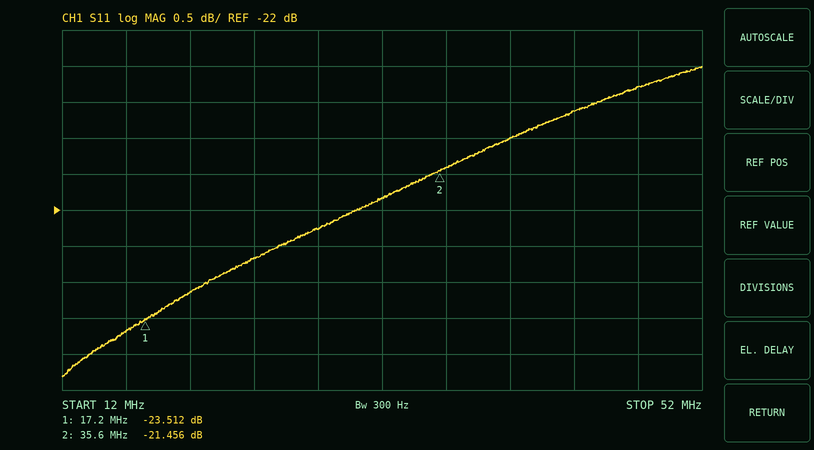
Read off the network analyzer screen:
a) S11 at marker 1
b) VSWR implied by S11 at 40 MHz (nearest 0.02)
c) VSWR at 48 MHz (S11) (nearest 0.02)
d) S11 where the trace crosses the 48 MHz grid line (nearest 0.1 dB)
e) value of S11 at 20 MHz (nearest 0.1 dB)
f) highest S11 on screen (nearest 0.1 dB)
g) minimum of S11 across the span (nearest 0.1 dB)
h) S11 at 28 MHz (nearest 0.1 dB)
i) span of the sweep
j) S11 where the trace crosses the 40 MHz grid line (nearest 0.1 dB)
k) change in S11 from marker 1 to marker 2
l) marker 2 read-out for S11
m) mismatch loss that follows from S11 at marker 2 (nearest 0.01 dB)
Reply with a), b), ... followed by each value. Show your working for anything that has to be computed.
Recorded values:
a) -23.512 dB
b) |Γ| = 10^(-21/20) = 0.0891; VSWR = (1 + 0.0891)/(1 − 0.0891) ≈ 1.20
c) |Γ| = 10^(-20.3/20) = 0.0966; VSWR = (1 + 0.0966)/(1 − 0.0966) ≈ 1.21, so 1.22 to the nearest 0.02
d) -20.3 dB
e) -23.1 dB
f) -20.0 dB
g) -24.3 dB
h) -22.3 dB
i) 40 MHz
j) -21.0 dB
k) -21.456 − (-23.512) = 2.056 dB
l) -21.456 dB
m) −10 log10(1 − 10^(-21.456/10)) ≈ 0.03 dB
